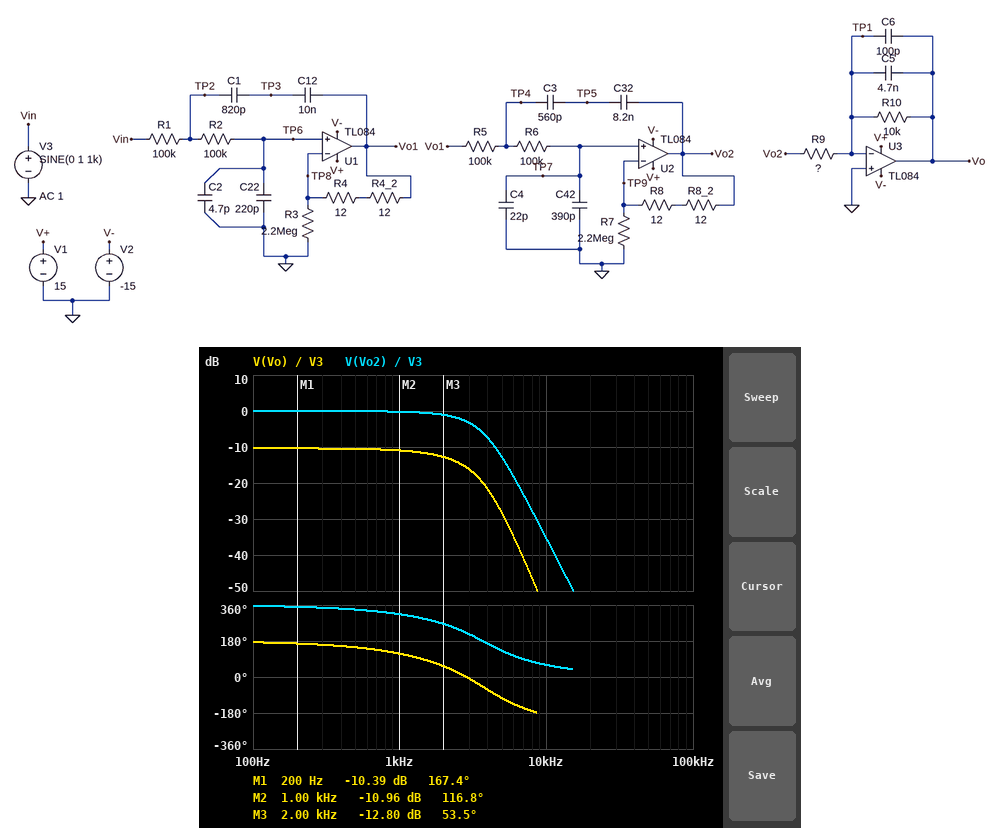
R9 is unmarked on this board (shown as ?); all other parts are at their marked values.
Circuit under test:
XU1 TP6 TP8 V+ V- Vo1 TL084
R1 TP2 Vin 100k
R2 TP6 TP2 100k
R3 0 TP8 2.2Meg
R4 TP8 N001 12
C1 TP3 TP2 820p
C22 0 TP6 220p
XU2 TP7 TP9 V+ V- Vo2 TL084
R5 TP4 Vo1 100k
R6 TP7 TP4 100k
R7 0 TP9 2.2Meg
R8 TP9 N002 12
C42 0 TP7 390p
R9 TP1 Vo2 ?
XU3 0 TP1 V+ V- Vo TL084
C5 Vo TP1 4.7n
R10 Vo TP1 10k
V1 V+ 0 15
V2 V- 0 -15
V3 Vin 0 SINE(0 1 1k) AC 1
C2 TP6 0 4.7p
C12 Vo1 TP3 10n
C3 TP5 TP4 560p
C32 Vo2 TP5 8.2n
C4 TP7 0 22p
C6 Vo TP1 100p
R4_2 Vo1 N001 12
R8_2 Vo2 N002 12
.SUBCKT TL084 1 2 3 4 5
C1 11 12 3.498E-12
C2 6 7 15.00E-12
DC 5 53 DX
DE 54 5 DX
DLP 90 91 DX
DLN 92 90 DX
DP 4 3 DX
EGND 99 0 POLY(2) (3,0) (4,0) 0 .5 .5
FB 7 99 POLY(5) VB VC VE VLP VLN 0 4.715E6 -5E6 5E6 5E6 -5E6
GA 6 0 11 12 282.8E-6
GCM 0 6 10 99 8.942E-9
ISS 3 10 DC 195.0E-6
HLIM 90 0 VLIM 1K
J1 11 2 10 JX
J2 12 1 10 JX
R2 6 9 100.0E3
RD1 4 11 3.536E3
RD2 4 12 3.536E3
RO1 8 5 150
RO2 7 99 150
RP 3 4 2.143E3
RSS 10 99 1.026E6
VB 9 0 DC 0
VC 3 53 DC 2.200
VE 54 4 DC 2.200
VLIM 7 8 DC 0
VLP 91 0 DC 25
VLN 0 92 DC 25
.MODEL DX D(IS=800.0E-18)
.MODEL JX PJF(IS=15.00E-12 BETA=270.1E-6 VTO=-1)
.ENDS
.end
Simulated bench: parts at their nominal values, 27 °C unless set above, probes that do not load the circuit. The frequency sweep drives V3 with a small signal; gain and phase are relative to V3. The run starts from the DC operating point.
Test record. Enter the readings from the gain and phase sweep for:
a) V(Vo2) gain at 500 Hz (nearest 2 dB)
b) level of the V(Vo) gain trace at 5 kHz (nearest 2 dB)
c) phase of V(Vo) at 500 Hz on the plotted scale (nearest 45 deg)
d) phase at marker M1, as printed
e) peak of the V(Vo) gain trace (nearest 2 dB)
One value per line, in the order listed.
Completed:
0 dB
-28 dB
135 deg
167.4 deg
-10 dB
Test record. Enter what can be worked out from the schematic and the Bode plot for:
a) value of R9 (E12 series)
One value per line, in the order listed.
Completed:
33 kΩ
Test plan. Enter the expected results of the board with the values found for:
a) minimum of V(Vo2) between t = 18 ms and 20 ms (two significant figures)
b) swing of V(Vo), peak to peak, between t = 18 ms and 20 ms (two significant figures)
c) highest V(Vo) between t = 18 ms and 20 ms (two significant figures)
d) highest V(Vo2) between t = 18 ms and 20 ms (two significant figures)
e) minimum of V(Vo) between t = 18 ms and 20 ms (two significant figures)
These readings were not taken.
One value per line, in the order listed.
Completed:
-980 mV
570 mV
280 mV
980 mV
-280 mV
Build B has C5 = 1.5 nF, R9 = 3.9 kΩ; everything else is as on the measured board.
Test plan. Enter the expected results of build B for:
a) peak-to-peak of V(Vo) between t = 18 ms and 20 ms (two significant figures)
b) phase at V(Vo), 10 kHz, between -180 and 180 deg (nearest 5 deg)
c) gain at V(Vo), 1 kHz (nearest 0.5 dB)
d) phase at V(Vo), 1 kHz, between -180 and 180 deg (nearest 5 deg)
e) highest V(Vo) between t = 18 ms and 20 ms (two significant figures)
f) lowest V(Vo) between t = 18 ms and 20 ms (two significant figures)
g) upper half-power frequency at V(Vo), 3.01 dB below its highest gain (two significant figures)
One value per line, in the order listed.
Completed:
5.0 V
-165 deg
8.0 dB
130 deg
2.5 V
-2.5 V
2.8 kHz
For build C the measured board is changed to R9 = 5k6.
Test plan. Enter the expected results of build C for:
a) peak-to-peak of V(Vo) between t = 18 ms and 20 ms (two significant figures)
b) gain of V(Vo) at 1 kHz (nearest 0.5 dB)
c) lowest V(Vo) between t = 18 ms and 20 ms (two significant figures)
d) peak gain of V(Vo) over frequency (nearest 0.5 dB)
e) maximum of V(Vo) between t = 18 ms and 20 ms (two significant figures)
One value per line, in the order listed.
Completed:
3.3 V
4.5 dB
-1.7 V
5.0 dB
1.7 V
